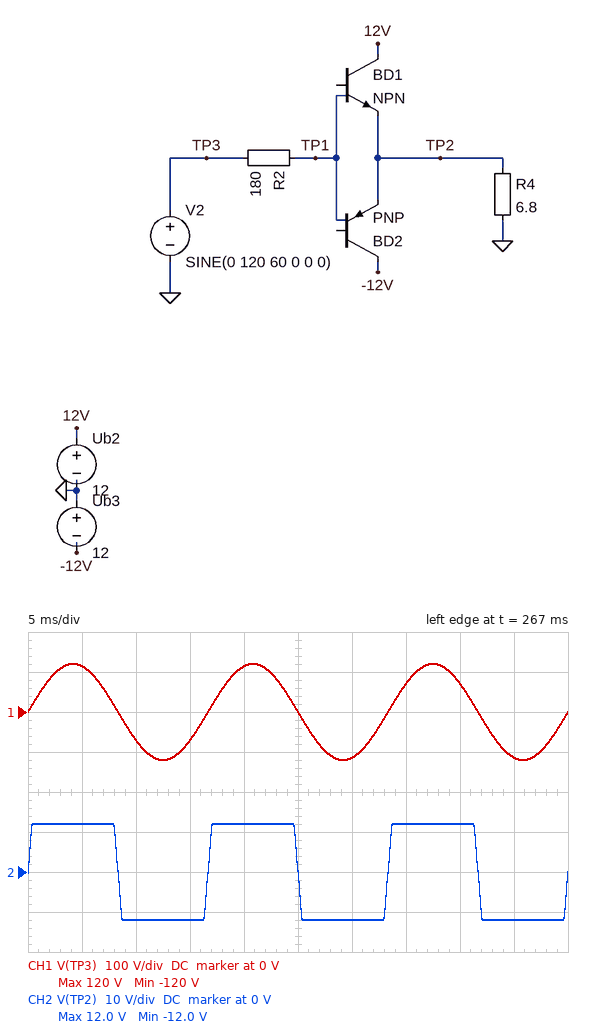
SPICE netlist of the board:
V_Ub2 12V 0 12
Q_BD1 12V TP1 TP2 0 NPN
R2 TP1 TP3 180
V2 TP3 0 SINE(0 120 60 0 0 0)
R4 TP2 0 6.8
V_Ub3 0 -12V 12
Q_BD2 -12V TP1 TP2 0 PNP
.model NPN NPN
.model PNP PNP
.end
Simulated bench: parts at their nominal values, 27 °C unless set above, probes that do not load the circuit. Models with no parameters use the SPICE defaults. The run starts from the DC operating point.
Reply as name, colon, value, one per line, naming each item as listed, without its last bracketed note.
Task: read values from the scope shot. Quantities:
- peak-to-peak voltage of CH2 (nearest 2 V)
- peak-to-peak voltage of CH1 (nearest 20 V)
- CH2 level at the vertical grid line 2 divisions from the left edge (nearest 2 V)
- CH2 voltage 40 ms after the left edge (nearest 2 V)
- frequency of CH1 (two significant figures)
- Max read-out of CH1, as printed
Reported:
peak-to-peak voltage of CH2: 24 V
peak-to-peak voltage of CH1: 240 V
CH2 level at the vertical grid line 2 divisions from the left edge: -12 V
CH2 voltage 40 ms after the left edge: 12 V
frequency of CH1: 60 Hz
Max read-out of CH1, as printed: 120 V
